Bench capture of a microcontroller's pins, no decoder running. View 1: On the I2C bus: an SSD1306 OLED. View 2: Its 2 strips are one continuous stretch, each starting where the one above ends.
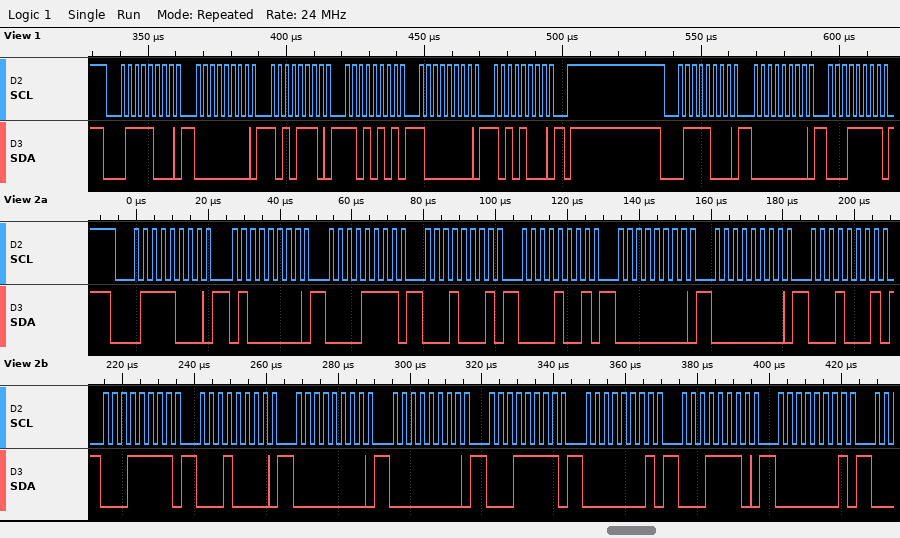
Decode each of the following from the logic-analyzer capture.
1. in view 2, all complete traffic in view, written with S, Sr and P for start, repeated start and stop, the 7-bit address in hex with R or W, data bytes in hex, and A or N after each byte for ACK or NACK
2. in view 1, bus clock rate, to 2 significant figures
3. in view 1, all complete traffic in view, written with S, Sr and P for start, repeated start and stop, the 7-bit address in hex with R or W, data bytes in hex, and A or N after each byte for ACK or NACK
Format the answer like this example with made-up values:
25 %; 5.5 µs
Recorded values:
S 3CW A 40 A 0F A 11 A 09 A 00 A 00 A 11 A 1F A 10 A 00 A 00 A 1F A 01 A 1E A 01 A; 400 kHz; S 3CW A 00 A AE A D5 A 80 A A8 A P S 3CW A 00 A 1F A
